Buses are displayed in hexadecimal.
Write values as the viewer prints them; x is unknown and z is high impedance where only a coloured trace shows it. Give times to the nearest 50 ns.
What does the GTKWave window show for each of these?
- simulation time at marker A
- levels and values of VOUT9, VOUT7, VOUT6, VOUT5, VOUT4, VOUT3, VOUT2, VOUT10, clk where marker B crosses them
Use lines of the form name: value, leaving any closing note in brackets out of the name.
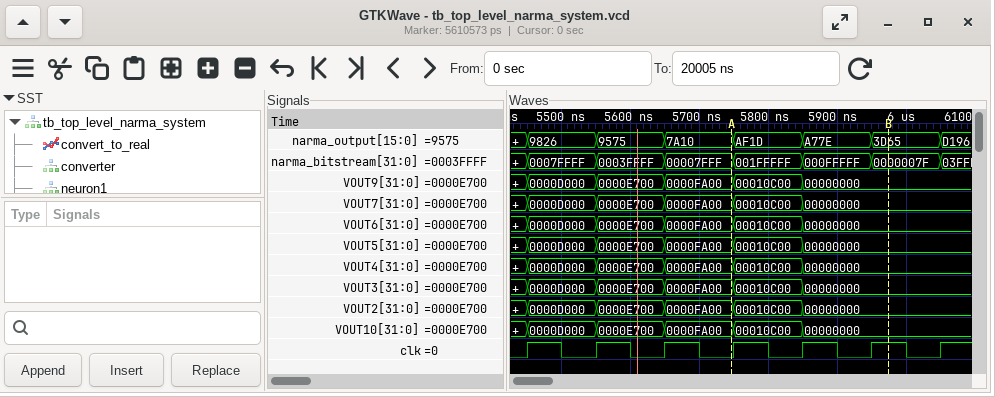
simulation time at marker A: 5750 ns
levels and values of VOUT9, VOUT7, VOUT6, VOUT5, VOUT4, VOUT3, VOUT2, VOUT10, clk where marker B crosses them: VOUT9=00000000, VOUT7=00000000, VOUT6=00000000, VOUT5=00000000, VOUT4=00000000, VOUT3=00000000, VOUT2=00000000, VOUT10=00000000, clk=1
